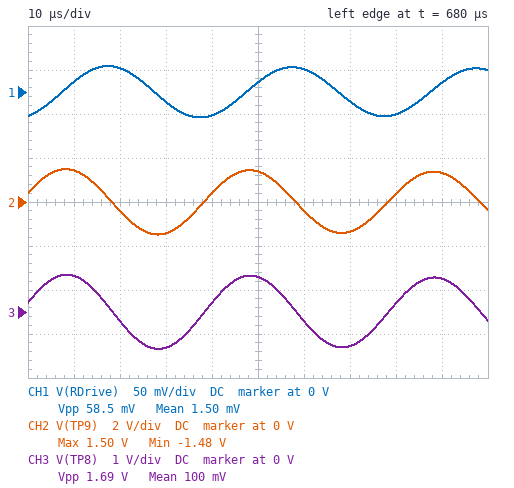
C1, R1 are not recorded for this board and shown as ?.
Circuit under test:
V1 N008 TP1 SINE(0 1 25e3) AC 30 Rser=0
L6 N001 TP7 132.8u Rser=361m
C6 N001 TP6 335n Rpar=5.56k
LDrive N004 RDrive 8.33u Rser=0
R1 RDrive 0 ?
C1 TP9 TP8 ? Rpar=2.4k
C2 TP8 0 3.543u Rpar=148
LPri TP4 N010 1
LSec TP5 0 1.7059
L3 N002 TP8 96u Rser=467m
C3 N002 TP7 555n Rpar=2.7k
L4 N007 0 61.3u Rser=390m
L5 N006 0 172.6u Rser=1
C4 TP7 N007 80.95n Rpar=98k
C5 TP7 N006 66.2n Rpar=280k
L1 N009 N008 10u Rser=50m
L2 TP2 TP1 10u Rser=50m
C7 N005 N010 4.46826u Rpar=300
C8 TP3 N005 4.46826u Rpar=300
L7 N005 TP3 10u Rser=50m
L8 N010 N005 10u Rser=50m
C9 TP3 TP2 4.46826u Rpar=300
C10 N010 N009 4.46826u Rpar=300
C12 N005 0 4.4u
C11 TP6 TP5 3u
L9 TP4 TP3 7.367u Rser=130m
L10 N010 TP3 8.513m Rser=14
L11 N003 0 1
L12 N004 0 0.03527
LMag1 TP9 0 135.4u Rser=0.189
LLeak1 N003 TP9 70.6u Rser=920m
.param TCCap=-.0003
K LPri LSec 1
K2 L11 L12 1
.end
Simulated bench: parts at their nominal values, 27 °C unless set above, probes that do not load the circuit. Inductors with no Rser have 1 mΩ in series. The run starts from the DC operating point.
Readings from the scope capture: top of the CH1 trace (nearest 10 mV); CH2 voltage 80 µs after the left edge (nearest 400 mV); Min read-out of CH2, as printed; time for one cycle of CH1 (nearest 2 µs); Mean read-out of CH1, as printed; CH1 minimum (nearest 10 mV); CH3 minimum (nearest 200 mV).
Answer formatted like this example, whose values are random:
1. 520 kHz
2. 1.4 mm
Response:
1. 30 mV
2. 400 mV
3. -1.48 V
4. 40 µs
5. 1.50 mV
6. -30 mV
7. -800 mV
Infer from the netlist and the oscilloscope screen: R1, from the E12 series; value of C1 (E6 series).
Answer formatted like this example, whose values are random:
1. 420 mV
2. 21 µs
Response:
1. 0.18 Ω
2. 1 µF
